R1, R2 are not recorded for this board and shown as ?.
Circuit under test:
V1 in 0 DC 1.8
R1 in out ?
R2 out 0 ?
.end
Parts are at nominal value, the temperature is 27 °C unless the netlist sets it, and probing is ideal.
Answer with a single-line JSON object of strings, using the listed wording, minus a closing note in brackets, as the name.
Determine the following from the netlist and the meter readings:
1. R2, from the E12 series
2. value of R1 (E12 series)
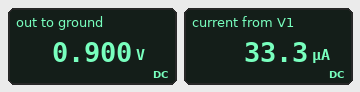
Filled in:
{"R2, from the E12 series": "27 kΩ", "value of R1": "27 kΩ"}
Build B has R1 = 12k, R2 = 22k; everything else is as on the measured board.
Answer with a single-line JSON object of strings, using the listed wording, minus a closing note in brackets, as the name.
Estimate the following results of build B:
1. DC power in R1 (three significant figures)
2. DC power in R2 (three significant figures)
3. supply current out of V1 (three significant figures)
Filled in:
{"DC power in R1": "33.6 µW", "DC power in R2": "61.7 µW", "supply current out of V1": "52.9 µA"}
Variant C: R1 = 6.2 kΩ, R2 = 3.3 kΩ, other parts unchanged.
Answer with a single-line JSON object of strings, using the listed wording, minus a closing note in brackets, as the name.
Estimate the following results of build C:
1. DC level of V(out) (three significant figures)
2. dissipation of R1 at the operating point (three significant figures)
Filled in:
{"DC level of V(out)": "625 mV", "dissipation of R1 at the operating point": "223 µW"}
